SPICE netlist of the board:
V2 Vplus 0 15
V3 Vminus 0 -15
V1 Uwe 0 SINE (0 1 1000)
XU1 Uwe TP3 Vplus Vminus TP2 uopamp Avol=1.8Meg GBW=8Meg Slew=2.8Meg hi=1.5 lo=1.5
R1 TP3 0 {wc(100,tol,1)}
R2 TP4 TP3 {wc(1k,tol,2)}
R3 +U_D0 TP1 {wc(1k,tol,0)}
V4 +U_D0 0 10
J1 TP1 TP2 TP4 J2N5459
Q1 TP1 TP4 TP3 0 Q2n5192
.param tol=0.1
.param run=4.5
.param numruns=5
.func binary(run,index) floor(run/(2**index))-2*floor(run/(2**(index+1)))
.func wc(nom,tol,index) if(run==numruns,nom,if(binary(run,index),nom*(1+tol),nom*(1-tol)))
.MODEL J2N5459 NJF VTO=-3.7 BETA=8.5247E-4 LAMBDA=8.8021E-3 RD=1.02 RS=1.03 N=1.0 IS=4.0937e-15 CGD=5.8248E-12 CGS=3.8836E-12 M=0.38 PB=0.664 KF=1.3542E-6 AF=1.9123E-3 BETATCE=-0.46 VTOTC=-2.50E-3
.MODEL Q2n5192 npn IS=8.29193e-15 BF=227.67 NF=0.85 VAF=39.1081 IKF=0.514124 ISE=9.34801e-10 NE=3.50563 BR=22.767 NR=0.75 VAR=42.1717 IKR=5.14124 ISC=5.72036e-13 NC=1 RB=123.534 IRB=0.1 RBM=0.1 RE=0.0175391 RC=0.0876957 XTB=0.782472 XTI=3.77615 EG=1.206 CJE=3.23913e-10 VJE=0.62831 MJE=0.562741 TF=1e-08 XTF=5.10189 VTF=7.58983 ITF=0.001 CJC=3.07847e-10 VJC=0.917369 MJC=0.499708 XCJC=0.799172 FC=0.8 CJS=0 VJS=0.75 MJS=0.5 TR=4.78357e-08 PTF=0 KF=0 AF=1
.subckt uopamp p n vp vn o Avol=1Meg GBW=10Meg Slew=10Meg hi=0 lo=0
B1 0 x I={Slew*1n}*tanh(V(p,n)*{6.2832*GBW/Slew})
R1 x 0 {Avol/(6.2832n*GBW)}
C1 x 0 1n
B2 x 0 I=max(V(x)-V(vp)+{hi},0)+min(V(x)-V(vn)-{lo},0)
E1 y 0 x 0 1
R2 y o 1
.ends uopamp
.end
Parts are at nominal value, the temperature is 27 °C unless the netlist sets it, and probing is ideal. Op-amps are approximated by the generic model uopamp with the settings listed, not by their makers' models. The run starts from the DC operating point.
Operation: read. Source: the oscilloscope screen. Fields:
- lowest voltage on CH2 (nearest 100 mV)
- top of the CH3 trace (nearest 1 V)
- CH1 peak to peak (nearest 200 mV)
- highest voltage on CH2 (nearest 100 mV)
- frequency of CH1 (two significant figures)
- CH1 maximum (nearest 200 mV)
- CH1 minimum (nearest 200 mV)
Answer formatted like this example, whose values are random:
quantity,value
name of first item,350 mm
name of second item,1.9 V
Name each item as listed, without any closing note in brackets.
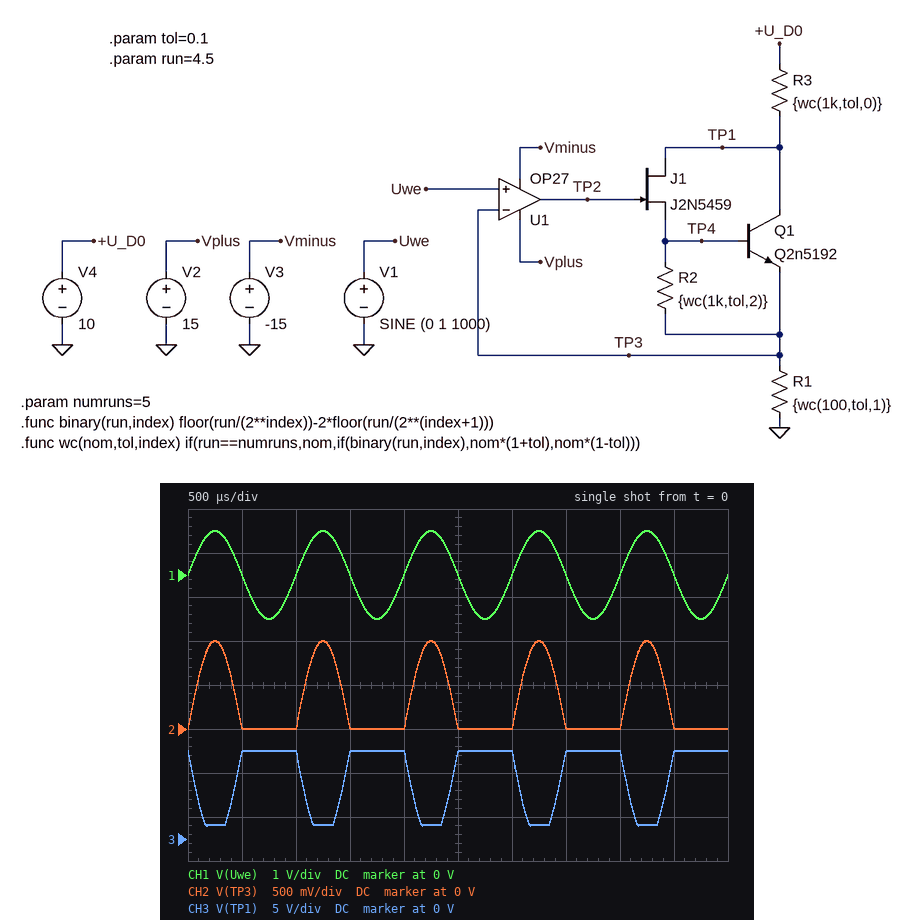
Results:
quantity,value
lowest voltage on CH2,0 V
top of the CH3 trace,10 V
CH1 peak to peak,2.0 V
highest voltage on CH2,1.0 V
frequency of CH1,1.0 kHz
CH1 maximum,1.0 V
CH1 minimum,-1.0 V
